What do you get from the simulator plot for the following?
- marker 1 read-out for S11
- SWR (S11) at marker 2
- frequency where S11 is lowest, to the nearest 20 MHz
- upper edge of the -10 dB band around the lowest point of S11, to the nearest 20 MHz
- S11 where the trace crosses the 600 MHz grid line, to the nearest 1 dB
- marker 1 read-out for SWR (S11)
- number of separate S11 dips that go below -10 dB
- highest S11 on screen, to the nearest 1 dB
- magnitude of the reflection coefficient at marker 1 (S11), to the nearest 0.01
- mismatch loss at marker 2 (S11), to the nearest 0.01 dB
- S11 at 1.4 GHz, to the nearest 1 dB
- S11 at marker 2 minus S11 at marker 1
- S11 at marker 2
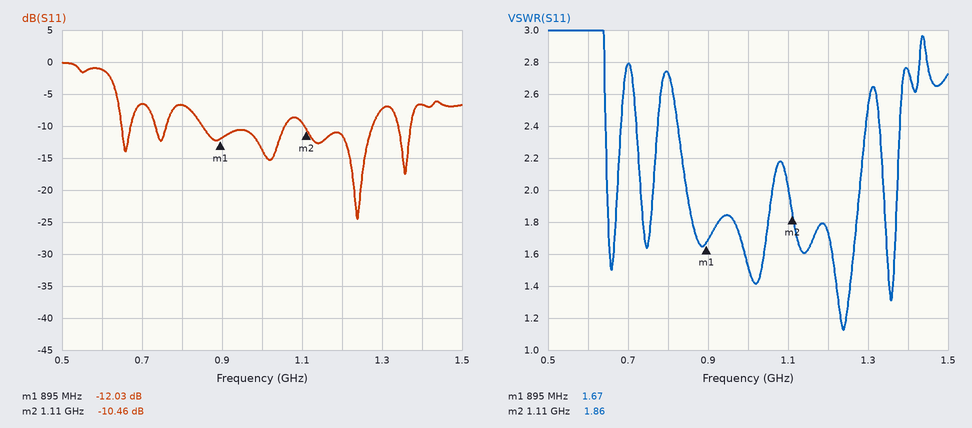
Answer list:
-12.03 dB
1.86
1.24 GHz
1.28 GHz
-1 dB
1.67
5
0 dB
0.25
0.41 dB
-7 dB
1.57 dB
-10.46 dB
